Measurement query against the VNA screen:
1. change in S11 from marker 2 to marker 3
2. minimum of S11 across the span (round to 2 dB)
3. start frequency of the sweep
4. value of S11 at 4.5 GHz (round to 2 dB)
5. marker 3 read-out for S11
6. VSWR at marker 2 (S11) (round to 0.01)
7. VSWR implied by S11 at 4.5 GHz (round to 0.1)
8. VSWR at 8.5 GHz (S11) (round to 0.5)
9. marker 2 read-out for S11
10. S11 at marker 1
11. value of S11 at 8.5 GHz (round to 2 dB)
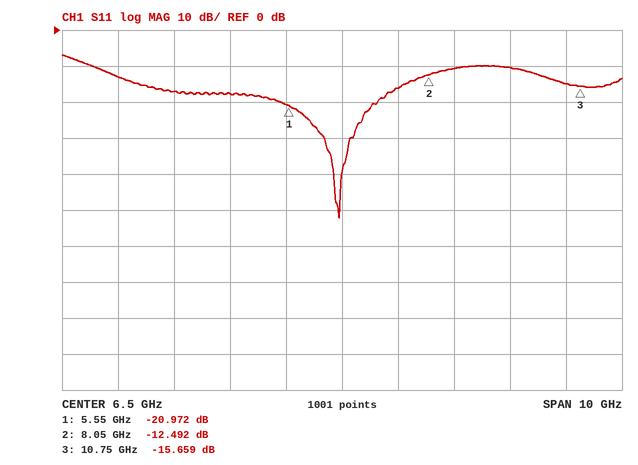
-3.167 dB
-52 dB
1.5 GHz
-18 dB
-15.659 dB
1.62
1.3
2.0
-12.492 dB
-20.972 dB
-10 dB
